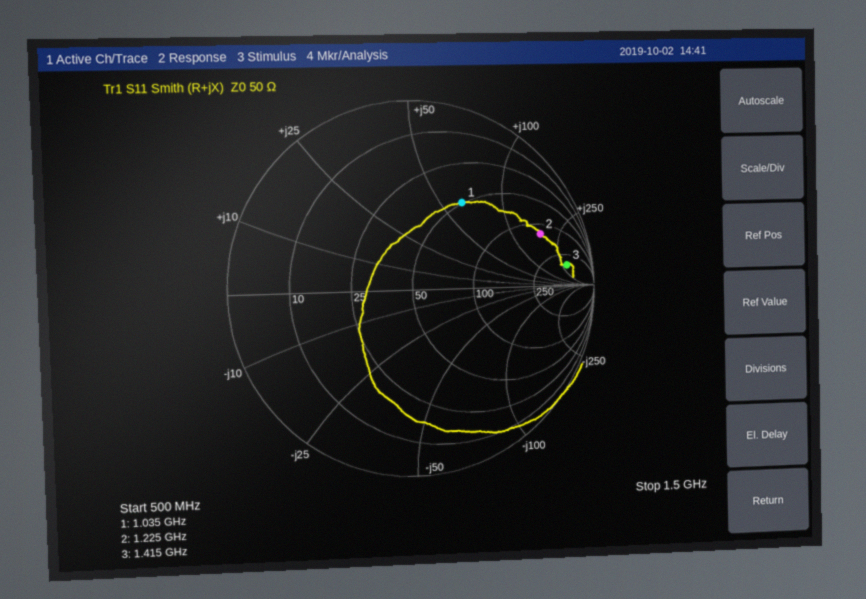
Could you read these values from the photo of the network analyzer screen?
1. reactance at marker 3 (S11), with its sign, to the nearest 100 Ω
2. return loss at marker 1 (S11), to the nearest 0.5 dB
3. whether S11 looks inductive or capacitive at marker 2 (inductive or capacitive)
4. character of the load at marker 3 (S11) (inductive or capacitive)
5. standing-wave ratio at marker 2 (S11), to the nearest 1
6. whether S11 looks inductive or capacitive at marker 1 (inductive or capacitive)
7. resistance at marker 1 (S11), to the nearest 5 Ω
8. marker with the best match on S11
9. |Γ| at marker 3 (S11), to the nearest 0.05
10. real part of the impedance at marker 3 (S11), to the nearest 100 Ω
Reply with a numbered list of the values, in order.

1. +300 Ω
2. 5.5 dB
3. inductive
4. inductive
5. 7
6. inductive
7. 50 Ω
8. marker 1
9. 0.85
10. 400 Ω
